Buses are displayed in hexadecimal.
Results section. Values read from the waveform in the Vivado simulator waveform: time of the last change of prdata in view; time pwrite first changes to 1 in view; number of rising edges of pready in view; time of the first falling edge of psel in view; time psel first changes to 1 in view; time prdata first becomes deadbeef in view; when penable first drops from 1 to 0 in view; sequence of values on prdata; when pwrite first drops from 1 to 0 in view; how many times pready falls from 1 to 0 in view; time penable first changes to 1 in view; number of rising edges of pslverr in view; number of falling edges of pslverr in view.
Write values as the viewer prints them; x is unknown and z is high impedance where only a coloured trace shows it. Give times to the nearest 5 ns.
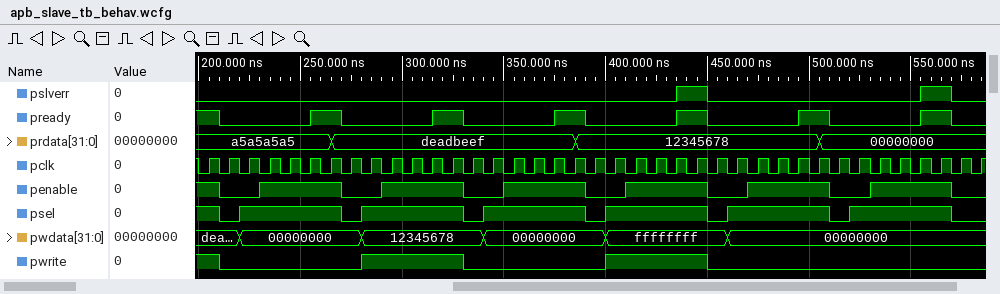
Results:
505 ns
280 ns
6
210 ns
220 ns
265 ns
210 ns
a5a5a5a5, deadbeef, 12345678, 00000000
210 ns
7
230 ns
2
2
